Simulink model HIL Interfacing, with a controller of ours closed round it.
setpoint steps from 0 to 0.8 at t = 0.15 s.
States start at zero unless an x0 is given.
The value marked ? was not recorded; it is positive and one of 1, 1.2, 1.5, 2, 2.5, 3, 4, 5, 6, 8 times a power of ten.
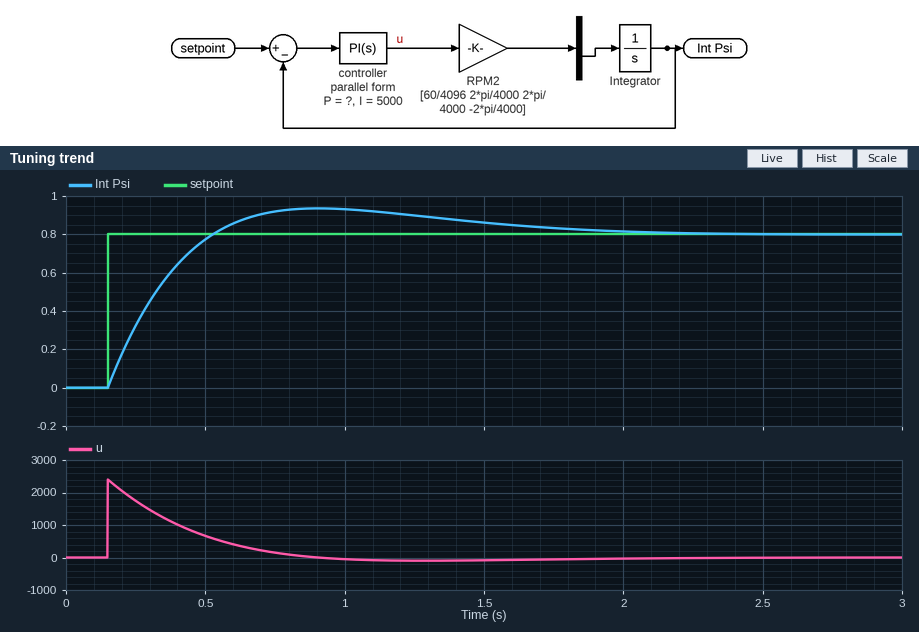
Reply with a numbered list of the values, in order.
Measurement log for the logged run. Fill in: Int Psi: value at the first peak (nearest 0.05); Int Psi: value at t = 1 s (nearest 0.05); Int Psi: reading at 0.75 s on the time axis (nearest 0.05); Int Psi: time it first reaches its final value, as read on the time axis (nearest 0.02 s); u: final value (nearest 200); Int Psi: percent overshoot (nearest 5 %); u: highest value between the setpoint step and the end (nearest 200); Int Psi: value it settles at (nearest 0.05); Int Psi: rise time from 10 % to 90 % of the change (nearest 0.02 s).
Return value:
1. 0.95
2. 0.95
3. 0.90
4. 0.52 s
5. 0
6. 15 %
7. 2400
8. 0.80
9. 0.28 s
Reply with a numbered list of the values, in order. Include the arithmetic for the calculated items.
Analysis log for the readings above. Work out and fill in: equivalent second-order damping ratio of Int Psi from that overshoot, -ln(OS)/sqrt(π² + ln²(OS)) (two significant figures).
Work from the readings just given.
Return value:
1. ln(0.15) = -1.897; 1.897 / sqrt(9.870 + 3.599) = 0.52
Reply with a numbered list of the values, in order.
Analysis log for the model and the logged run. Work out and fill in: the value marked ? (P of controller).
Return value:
1. 3000
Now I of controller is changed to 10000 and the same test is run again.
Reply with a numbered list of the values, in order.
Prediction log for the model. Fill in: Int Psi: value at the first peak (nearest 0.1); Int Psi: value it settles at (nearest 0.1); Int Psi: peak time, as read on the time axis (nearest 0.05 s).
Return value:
1. 1.0
2. 0.8
3. 0.75 s
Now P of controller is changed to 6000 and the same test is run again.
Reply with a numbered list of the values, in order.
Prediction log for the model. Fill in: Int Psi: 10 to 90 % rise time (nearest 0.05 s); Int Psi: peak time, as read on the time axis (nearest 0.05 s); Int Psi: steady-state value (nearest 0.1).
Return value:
1. 0.20 s
2. 0.75 s
3. 0.8
